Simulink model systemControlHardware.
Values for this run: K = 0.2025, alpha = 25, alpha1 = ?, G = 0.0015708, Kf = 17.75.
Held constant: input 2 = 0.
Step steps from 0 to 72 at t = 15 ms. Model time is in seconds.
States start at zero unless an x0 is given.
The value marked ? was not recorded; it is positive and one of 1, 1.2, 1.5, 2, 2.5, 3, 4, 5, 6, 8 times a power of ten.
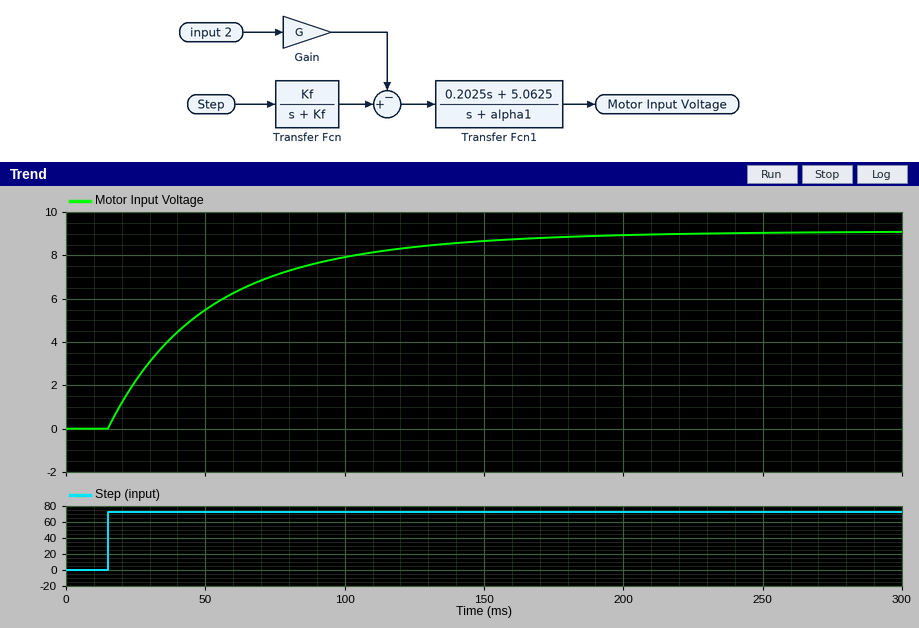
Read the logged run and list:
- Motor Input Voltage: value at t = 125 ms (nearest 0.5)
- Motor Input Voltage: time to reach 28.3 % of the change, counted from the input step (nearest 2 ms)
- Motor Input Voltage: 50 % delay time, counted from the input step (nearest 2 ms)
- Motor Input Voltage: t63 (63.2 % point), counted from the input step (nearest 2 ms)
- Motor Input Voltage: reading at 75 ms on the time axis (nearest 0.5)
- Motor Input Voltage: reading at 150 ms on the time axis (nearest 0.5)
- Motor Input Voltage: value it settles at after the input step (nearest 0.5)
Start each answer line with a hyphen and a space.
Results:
- 8.5
- 12 ms
- 26 ms
- 38 ms
- 7.0
- 8.5
- 9.0
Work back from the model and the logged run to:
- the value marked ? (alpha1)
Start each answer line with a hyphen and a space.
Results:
- 40
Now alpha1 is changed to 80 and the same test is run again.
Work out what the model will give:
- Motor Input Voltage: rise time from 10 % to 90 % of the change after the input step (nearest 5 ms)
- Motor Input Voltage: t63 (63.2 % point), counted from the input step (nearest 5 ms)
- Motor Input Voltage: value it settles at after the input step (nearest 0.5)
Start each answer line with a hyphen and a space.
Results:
- 75 ms
- 20 ms
- 4.5
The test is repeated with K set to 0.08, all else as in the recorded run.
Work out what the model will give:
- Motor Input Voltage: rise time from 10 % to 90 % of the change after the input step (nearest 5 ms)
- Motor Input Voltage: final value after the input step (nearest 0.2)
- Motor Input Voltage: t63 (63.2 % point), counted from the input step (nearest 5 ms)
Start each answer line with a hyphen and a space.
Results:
- 95 ms
- 3.6
- 40 ms
